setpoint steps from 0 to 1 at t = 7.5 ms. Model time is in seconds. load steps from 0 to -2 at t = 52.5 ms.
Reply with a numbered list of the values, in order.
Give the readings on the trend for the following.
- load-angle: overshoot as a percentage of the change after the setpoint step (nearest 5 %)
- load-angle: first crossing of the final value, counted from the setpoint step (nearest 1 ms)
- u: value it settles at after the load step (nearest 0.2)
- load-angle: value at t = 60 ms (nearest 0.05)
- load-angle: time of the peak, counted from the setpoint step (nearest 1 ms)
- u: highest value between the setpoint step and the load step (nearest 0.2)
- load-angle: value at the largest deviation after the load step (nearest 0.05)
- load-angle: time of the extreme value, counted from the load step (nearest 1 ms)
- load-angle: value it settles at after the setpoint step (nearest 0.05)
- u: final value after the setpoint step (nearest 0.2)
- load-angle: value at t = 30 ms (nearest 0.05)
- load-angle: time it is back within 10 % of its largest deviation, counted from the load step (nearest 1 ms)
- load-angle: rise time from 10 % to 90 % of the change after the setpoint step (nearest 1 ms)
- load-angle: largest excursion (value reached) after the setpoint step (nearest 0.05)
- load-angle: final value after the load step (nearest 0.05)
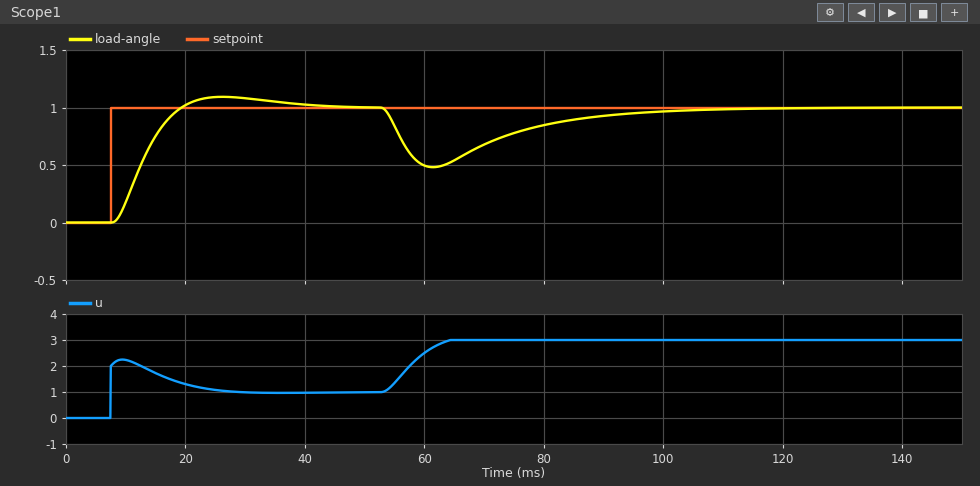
1. 10 %
2. 12 ms
3. 3.0
4. 0.50
5. 19 ms
6. 2.2
7. 0.50
8. 9 ms
9. 1.00
10. 1.0
11. 1.10
12. 42 ms
13. 8 ms
14. 1.10
15. 1.00
